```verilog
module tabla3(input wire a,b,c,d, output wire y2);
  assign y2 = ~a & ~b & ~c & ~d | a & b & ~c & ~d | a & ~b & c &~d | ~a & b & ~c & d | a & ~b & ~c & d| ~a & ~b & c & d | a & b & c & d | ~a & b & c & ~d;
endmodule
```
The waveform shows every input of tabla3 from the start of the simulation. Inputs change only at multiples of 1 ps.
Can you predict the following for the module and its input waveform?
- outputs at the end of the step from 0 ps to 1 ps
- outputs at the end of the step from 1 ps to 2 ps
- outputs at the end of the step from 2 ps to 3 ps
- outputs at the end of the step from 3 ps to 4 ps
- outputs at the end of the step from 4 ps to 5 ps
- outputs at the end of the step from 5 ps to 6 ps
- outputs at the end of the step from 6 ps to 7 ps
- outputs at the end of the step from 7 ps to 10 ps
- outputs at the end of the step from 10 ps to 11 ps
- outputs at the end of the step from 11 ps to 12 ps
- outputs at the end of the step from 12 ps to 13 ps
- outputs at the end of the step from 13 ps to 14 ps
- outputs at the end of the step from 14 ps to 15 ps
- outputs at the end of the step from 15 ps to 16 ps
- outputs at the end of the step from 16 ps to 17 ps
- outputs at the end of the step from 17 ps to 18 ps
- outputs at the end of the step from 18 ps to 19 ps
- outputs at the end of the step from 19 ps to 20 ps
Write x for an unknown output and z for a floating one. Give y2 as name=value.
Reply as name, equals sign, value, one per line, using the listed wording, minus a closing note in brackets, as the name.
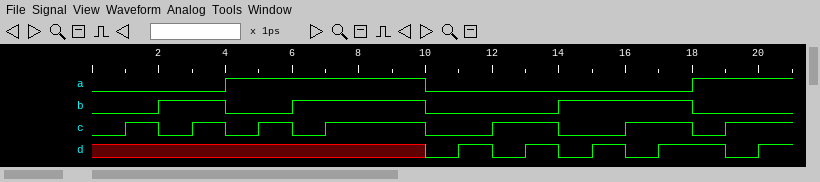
outputs at the end of the step from 0 ps to 1 ps = y2=x
outputs at the end of the step from 1 ps to 2 ps = y2=x
outputs at the end of the step from 2 ps to 3 ps = y2=x
outputs at the end of the step from 3 ps to 4 ps = y2=x
outputs at the end of the step from 4 ps to 5 ps = y2=x
outputs at the end of the step from 5 ps to 6 ps = y2=x
outputs at the end of the step from 6 ps to 7 ps = y2=x
outputs at the end of the step from 7 ps to 10 ps = y2=x
outputs at the end of the step from 10 ps to 11 ps = y2=1
outputs at the end of the step from 11 ps to 12 ps = y2=0
outputs at the end of the step from 12 ps to 13 ps = y2=0
outputs at the end of the step from 13 ps to 14 ps = y2=1
outputs at the end of the step from 14 ps to 15 ps = y2=0
outputs at the end of the step from 15 ps to 16 ps = y2=1
outputs at the end of the step from 16 ps to 17 ps = y2=1
outputs at the end of the step from 17 ps to 18 ps = y2=0
outputs at the end of the step from 18 ps to 19 ps = y2=1
outputs at the end of the step from 19 ps to 20 ps = y2=1
